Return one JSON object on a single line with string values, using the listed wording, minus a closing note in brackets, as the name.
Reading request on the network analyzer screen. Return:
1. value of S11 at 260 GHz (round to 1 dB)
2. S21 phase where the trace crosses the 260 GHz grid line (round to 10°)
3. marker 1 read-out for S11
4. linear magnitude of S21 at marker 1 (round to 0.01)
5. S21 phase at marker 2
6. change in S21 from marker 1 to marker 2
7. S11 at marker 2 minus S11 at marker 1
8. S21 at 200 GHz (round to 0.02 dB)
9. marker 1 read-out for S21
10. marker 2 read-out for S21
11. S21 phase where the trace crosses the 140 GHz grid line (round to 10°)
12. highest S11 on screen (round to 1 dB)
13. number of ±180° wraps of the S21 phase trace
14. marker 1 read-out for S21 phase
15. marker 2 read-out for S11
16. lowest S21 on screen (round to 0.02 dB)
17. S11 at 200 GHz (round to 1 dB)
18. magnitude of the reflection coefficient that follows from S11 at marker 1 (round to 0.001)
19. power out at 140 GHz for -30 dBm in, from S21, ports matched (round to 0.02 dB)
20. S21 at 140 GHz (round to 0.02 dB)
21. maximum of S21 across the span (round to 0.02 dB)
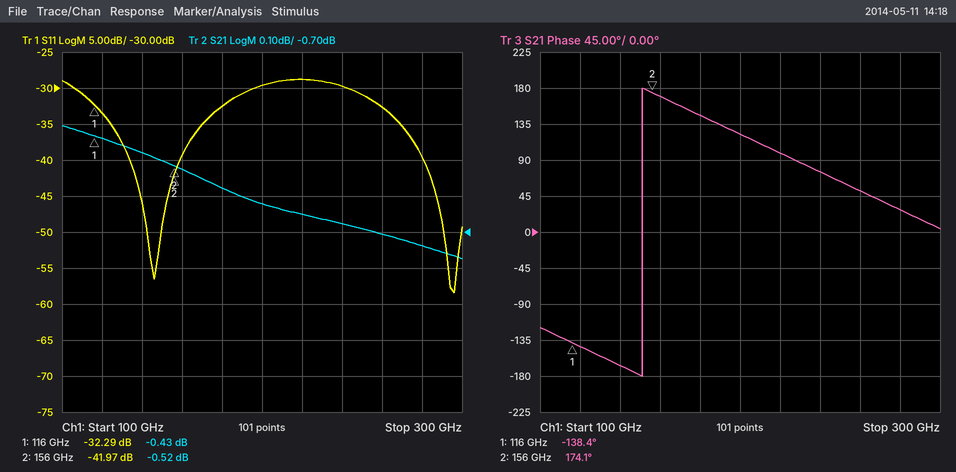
{"value of S11 at 260 GHz": "-33 dB", "S21 phase where the trace crosses the 260 GHz grid line": "50°", "marker 1 read-out for S11": "-32.29 dB", "linear magnitude of S21 at marker 1": "0.95", "S21 phase at marker 2": "174.1°", "change in S21 from marker 1 to marker 2": "-0.09 dB", "S11 at marker 2 minus S11 at marker 1": "-9.68 dB", "S21 at 200 GHz": "-0.62 dB", "marker 1 read-out for S21": "-0.43 dB", "marker 2 read-out for S21": "-0.52 dB", "S21 phase where the trace crosses the 140 GHz grid line": "-170°", "highest S11 on screen": "-29 dB", "number of ±180° wraps of the S21 phase trace": "1", "marker 1 read-out for S21 phase": "-138.4°", "marker 2 read-out for S11": "-41.97 dB", "lowest S21 on screen": "-0.78 dB", "S11 at 200 GHz": "-30 dB", "magnitude of the reflection coefficient that follows from S11 at marker 1": "0.024", "power out at 140 GHz for -30 dBm in, from S21, ports matched": "-30.48 dBm", "S21 at 140 GHz": "-0.48 dB", "maximum of S21 across the span": "-0.40 dB"}
